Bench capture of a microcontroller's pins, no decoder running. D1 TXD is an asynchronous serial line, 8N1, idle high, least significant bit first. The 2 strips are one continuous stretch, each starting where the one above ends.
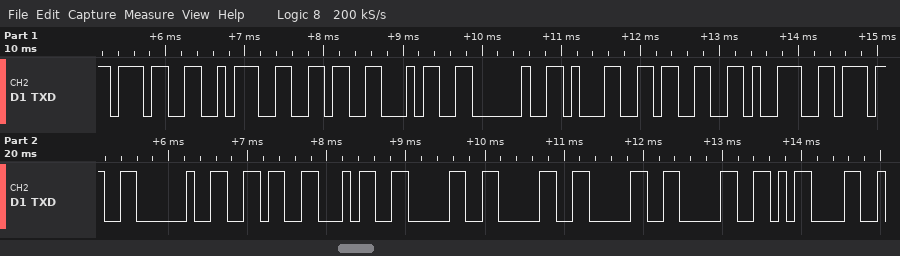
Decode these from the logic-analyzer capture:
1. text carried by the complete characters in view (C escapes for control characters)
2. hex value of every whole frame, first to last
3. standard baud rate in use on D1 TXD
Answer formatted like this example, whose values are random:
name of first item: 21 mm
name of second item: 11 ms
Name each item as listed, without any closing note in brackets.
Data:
text carried by the complete characters in view: "7:64 1397 640000\r"
hex value of every whole frame, first to last: 37 3A 36 34 20 31 33 39 37 20 36 34 30 30 30 30 0D
standard baud rate in use on D1 TXD: 9600 baud
